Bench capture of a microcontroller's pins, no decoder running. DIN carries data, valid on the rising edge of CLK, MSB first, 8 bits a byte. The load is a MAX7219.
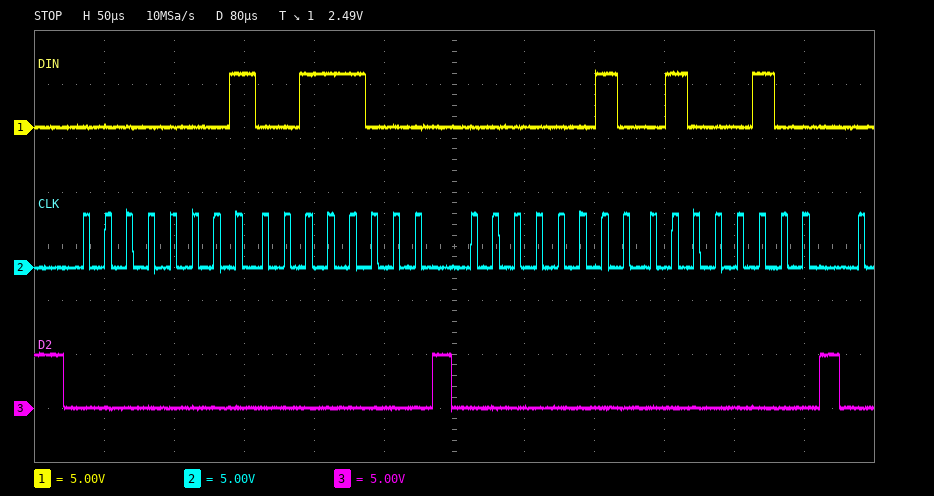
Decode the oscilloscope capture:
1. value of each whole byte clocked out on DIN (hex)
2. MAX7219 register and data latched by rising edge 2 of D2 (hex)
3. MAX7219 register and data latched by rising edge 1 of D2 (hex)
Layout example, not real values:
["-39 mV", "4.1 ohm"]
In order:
["01 38 02 44", "register 0x2, data 0x44", "register 0x1, data 0x38"]
